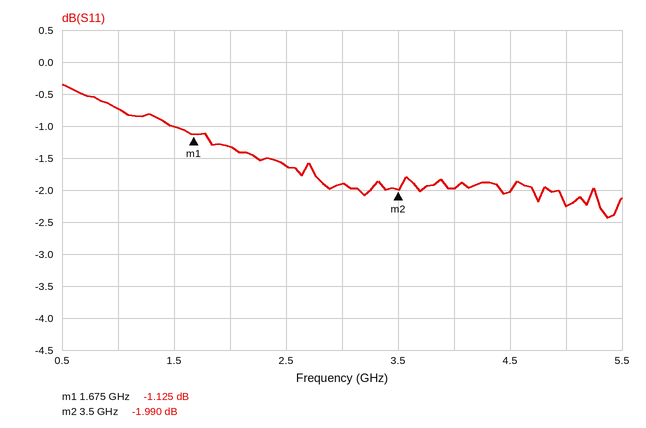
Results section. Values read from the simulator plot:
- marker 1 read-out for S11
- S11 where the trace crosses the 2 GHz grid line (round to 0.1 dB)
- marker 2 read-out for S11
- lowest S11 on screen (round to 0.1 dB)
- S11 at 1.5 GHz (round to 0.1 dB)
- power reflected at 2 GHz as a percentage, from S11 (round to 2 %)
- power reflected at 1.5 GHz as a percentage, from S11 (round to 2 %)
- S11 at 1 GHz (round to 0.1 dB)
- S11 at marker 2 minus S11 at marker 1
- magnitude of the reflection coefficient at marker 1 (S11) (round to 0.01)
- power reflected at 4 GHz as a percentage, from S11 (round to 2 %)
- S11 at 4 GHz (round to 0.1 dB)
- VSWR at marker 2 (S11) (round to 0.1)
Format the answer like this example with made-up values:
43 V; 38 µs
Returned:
-1.125 dB; -1.3 dB; -1.990 dB; -2.4 dB; -1.0 dB; 74 %; 80 %; -0.7 dB; -0.865 dB; 0.88; 64 %; -2.0 dB; 8.8
